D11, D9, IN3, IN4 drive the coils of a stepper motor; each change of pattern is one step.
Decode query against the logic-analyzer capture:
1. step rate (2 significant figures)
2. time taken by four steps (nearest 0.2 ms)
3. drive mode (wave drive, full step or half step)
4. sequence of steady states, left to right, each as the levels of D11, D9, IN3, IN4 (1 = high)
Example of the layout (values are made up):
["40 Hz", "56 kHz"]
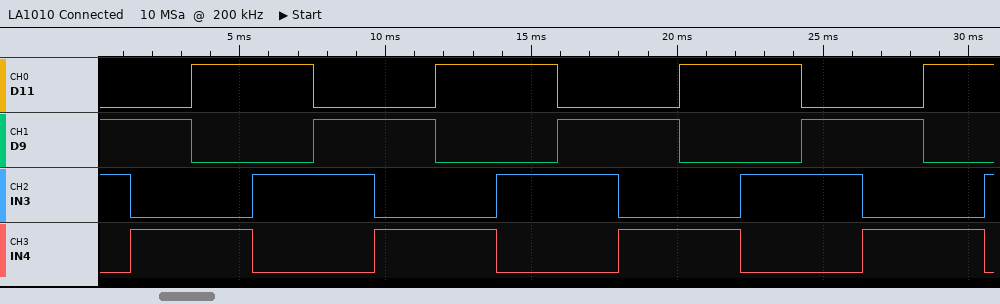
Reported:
["480 steps/s", "8.4 ms", "full step", "0110 0101 1001 1010 0110 0101 1001 1010 0110 0101 1001 1010 0110 0101 1001 1010"]
